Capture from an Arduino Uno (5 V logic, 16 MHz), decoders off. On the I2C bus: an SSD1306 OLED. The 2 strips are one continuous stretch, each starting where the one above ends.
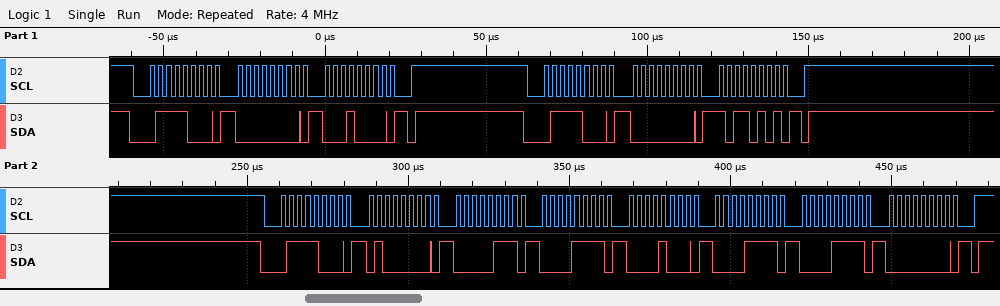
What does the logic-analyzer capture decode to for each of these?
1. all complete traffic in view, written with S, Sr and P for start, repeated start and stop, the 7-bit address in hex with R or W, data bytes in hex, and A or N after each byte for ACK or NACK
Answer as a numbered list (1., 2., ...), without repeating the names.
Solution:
1. S 3CW A 00 A 10 A P S 3CW A 00 A B5 A P S 3CW A 40 A 07 A 0F A 08 A 0F A 0F A 00 A P
